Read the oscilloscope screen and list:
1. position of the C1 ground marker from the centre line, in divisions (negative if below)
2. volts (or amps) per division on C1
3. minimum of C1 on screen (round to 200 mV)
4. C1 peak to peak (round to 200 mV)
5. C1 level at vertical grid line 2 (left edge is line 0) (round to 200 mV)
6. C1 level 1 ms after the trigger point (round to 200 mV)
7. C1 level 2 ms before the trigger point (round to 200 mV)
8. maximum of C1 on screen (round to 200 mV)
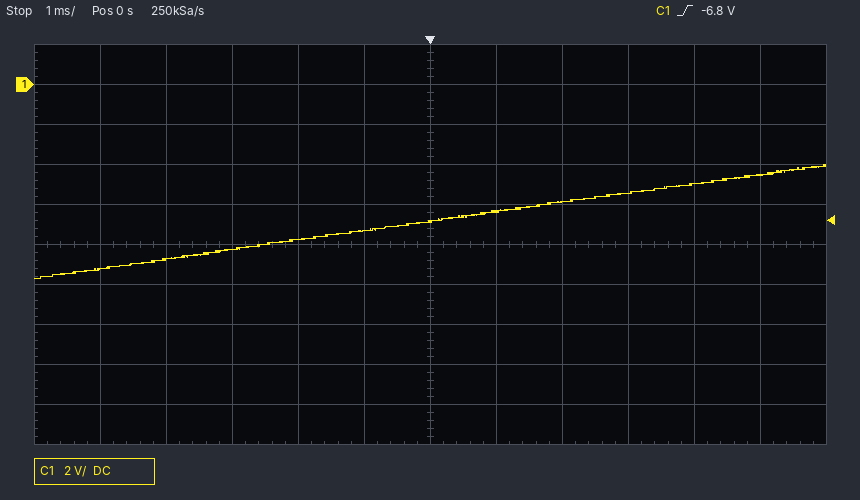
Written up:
+4.0 div
2 V
-9.6 V
5.6 V
-8.8 V
-6.4 V
-7.8 V
-4.0 V
